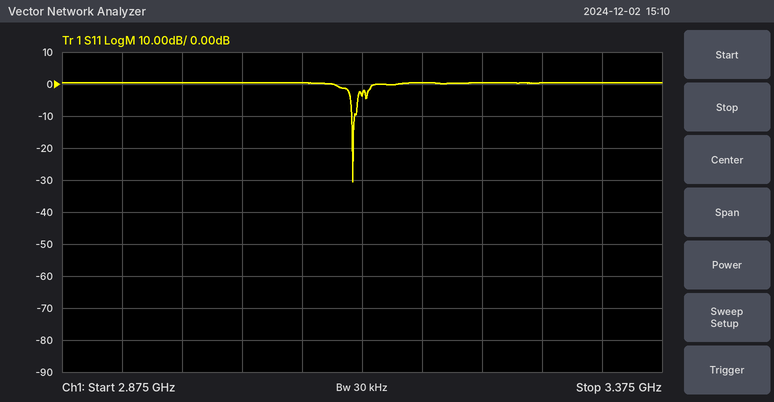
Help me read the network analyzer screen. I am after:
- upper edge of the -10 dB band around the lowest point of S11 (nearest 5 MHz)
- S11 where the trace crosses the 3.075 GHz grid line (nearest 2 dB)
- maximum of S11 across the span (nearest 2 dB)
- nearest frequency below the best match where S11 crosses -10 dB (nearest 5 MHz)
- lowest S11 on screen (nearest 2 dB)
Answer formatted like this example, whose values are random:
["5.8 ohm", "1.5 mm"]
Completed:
["3.120 GHz", "0 dB", "0 dB", "3.115 GHz", "-30 dB"]
